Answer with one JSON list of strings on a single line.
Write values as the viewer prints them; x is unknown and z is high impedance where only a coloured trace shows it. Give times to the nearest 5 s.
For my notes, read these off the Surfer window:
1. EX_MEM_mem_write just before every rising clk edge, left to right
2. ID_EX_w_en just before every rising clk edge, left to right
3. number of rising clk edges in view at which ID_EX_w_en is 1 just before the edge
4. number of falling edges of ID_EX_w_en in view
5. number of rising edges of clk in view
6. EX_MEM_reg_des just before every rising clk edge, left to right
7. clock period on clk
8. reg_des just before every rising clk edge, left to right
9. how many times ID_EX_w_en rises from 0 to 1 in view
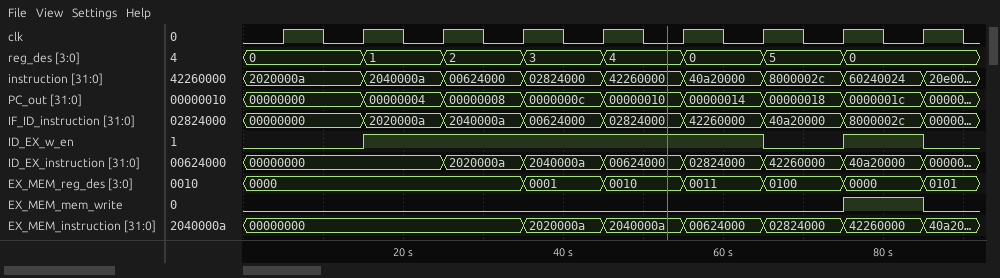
["0 0 0 0 0 0 0 0 1", "0 0 1 1 1 1 1 0 1", "6", "2", "9", "0000, 0000, 0000, 0000, 0001, 0010, 0011, 0100, 0000", "10 s", "0, 0, 1, 2, 3, 4, 0, 5, 0", "2"]
